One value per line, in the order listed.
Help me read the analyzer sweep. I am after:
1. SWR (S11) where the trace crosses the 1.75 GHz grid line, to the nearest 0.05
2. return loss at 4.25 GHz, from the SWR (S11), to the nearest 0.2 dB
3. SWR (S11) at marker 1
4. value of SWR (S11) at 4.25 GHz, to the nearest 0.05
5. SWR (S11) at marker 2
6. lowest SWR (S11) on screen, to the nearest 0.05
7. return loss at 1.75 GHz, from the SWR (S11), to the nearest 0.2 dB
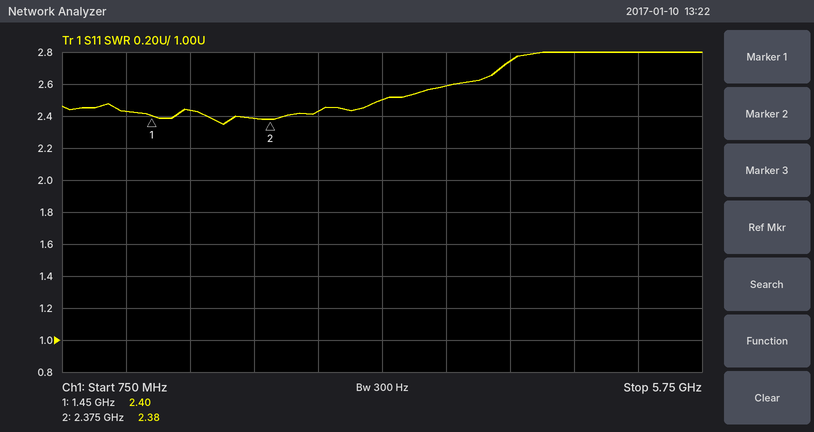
2.45
6.6 dB
2.40
2.75
2.38
2.35
7.6 dB
